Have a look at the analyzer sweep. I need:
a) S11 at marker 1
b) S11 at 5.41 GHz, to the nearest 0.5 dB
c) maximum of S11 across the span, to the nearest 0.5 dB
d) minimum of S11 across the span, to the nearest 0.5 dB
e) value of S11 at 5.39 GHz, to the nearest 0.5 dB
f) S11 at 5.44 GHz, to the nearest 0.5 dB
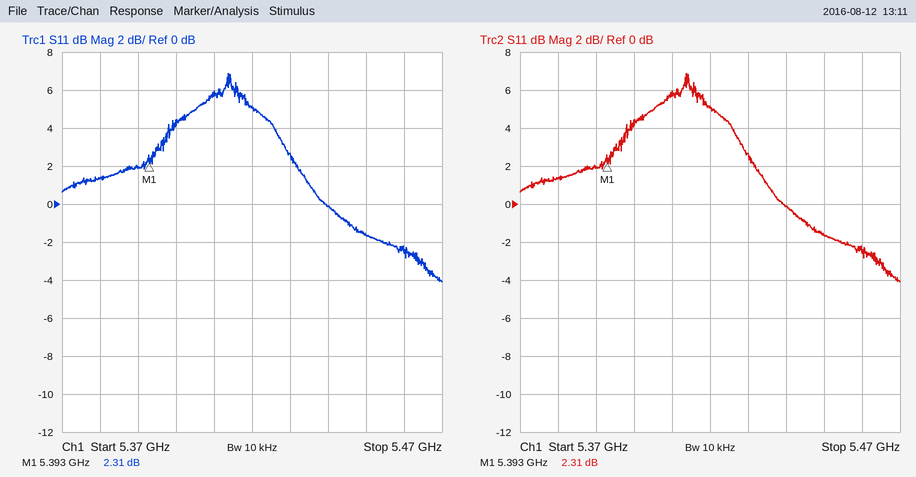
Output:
2.31 dB
6.0 dB
7.0 dB
-4.0 dB
2.0 dB
0.0 dB
